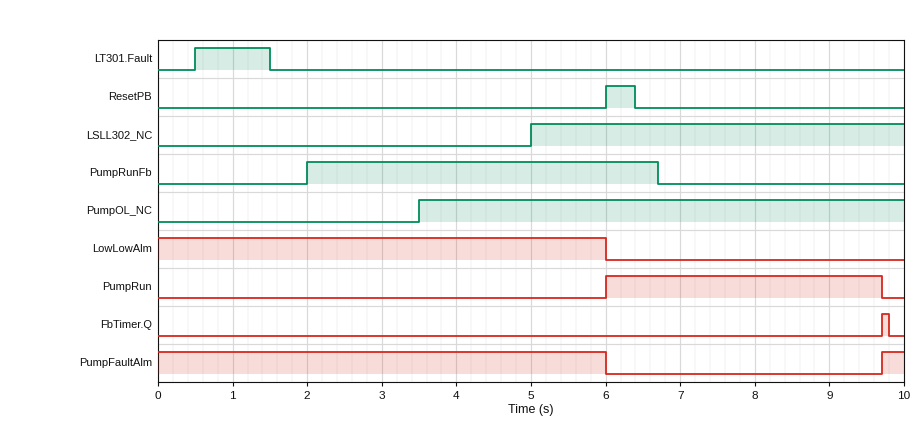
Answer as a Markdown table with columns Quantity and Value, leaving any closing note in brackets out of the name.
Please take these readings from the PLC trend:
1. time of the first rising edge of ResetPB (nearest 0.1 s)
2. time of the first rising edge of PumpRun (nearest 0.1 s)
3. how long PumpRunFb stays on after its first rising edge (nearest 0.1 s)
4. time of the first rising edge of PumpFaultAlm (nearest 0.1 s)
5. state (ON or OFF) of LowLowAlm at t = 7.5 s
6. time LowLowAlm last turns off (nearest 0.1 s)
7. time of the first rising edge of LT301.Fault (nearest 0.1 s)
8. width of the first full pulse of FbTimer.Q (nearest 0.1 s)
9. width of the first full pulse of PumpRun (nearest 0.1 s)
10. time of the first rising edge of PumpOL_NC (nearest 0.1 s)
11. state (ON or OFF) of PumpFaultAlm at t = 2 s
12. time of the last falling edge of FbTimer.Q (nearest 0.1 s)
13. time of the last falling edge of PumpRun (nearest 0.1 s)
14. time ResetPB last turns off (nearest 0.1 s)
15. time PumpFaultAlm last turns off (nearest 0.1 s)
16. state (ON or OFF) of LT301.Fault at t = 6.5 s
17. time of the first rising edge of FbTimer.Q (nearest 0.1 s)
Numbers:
| Quantity | Value |
|---|---|
| time of the first rising edge of ResetPB | 6.0 s |
| time of the first rising edge of PumpRun | 6.0 s |
| how long PumpRunFb stays on after its first rising edge | 4.7 s |
| time of the first rising edge of PumpFaultAlm | 9.7 s |
| state (ON or OFF) of LowLowAlm at t = 7.5 s | OFF |
| time LowLowAlm last turns off | 6.0 s |
| time of the first rising edge of LT301.Fault | 0.5 s |
| width of the first full pulse of FbTimer.Q | 0.1 s |
| width of the first full pulse of PumpRun | 3.7 s |
| time of the first rising edge of PumpOL_NC | 3.5 s |
| state (ON or OFF) of PumpFaultAlm at t = 2 s | ON |
| time of the last falling edge of FbTimer.Q | 9.8 s |
| time of the last falling edge of PumpRun | 9.7 s |
| time ResetPB last turns off | 6.4 s |
| time PumpFaultAlm last turns off | 6.0 s |
| state (ON or OFF) of LT301.Fault at t = 6.5 s | OFF |
| time of the first rising edge of FbTimer.Q | 9.7 s |
